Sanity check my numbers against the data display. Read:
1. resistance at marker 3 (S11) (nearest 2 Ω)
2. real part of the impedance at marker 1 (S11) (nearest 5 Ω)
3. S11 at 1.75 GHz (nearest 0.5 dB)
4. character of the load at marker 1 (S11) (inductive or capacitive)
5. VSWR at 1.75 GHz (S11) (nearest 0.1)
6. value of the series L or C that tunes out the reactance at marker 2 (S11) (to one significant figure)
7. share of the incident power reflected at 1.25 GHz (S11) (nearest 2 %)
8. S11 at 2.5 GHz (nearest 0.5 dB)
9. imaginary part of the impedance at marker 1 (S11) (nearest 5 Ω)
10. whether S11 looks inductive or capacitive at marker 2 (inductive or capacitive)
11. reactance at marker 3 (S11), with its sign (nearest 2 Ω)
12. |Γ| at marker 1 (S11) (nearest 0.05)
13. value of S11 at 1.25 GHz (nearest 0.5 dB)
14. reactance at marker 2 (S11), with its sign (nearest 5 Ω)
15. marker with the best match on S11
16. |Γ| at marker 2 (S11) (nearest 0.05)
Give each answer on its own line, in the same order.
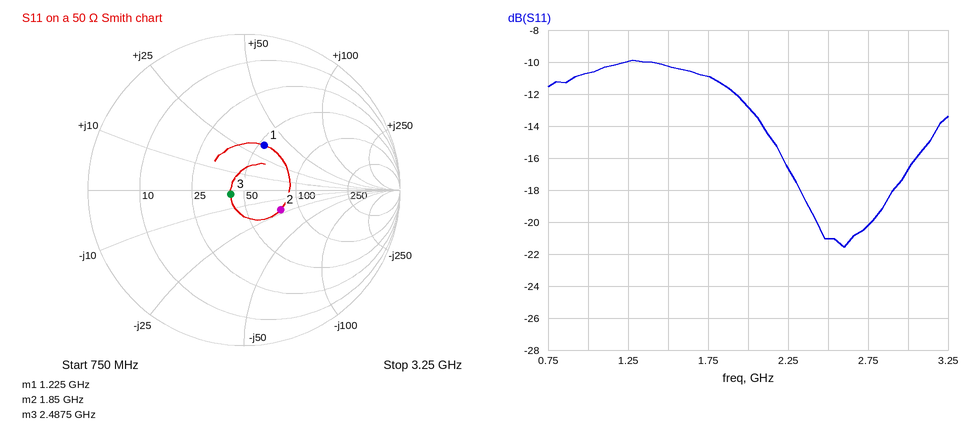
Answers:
42 Ω
55 Ω
-11.0 dB
inductive
1.8
2 nH
10 %
-21.0 dB
+35 Ω
capacitive
-2 Ω
0.30
-10.0 dB
-20 Ω
marker 3
0.25
